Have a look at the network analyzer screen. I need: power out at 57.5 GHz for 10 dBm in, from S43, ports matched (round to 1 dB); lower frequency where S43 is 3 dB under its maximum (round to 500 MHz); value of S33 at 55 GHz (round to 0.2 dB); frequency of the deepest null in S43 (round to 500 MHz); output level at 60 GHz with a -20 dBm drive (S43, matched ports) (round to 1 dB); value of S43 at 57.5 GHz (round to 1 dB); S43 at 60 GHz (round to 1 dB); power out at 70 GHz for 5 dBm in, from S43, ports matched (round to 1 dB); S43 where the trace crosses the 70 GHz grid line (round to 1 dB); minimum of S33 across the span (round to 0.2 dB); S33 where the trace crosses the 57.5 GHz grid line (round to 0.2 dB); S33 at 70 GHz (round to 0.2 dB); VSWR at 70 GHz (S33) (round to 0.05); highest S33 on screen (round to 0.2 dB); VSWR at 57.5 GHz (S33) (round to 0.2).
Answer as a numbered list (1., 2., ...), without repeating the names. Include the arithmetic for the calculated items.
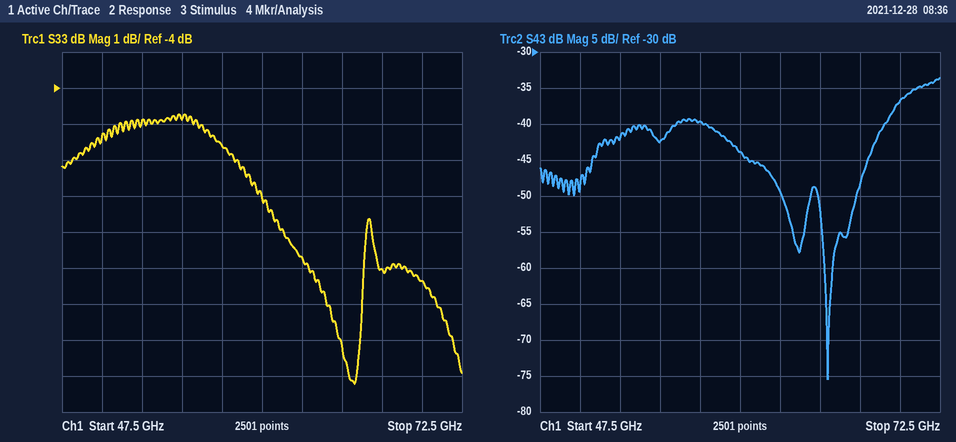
1. 10 dBm + (-40 dB) = -30 dBm
2. 70.0 GHz
3. -4.8 dB
4. 65.5 GHz
5. -20 dBm + (-44 dB) = -64 dBm
6. -40 dB
7. -44 dB
8. 5 dBm + (-37 dB) = -32 dBm
9. -37 dB
10. -12.2 dB
11. -5.6 dB
12. -9.4 dB
13. |Γ| = 10^(-9.4/20) = 0.3388; VSWR = (1 + 0.3388)/(1 − 0.3388) ≈ 2.03, so 2.05 to the nearest 0.05
14. -4.8 dB
15. |Γ| = 10^(-5.6/20) = 0.5248; VSWR = (1 + 0.5248)/(1 − 0.5248) ≈ 3.2
